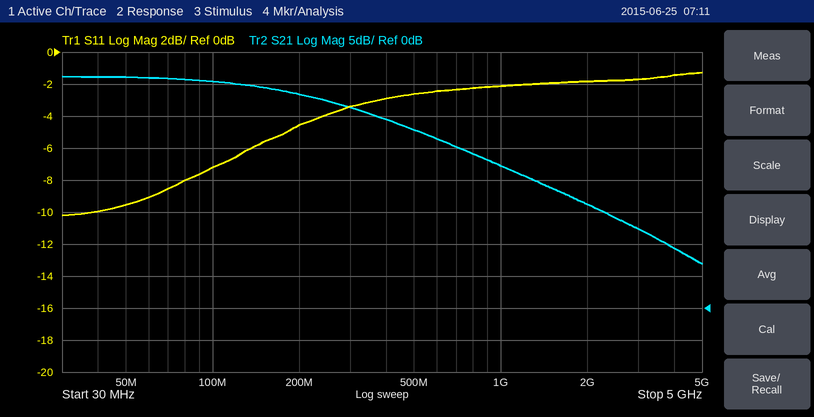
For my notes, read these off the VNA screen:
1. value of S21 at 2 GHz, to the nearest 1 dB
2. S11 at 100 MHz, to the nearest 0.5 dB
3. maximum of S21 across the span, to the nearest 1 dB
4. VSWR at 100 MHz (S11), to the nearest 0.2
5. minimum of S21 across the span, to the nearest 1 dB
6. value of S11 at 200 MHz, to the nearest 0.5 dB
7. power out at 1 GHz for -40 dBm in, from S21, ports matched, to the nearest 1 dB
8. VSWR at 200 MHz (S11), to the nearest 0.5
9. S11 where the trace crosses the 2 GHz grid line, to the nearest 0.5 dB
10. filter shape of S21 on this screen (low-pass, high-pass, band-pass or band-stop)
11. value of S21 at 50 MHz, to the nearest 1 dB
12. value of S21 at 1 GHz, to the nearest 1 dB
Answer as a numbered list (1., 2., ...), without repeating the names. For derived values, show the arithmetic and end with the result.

1. 16 dB
2. -7.0 dB
3. 36 dB
4. |Γ| = 10^(-7/20) = 0.4467; VSWR = (1 + 0.4467)/(1 − 0.4467) ≈ 2.6
5. 7 dB
6. -4.5 dB
7. -40 dBm + (22 dB) = -18 dBm
8. |Γ| = 10^(-4.5/20) = 0.5957; VSWR = (1 + 0.5957)/(1 − 0.5957) ≈ 4.0
9. -2.0 dB
10. low-pass
11. 36 dB
12. 22 dB
